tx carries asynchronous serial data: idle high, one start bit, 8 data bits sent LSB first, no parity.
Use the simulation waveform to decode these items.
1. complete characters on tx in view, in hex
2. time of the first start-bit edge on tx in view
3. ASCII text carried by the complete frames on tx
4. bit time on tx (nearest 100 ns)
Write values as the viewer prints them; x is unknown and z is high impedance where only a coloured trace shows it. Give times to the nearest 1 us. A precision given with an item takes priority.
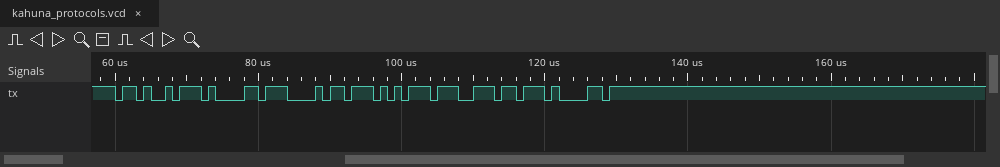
4B, 61, 68, 75, 6E, 61
60 us
"Kahuna"
1000 ns
